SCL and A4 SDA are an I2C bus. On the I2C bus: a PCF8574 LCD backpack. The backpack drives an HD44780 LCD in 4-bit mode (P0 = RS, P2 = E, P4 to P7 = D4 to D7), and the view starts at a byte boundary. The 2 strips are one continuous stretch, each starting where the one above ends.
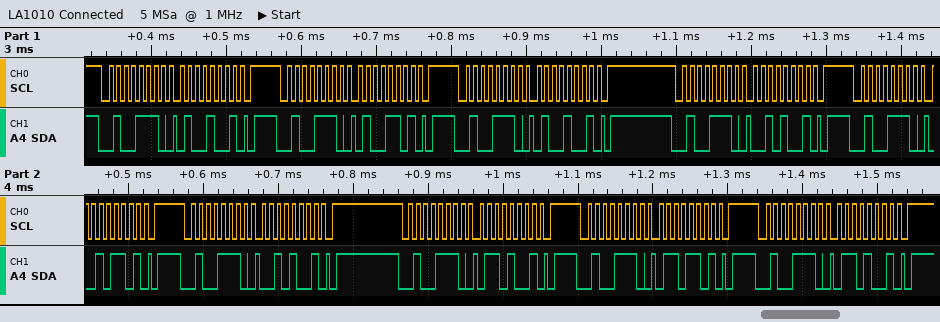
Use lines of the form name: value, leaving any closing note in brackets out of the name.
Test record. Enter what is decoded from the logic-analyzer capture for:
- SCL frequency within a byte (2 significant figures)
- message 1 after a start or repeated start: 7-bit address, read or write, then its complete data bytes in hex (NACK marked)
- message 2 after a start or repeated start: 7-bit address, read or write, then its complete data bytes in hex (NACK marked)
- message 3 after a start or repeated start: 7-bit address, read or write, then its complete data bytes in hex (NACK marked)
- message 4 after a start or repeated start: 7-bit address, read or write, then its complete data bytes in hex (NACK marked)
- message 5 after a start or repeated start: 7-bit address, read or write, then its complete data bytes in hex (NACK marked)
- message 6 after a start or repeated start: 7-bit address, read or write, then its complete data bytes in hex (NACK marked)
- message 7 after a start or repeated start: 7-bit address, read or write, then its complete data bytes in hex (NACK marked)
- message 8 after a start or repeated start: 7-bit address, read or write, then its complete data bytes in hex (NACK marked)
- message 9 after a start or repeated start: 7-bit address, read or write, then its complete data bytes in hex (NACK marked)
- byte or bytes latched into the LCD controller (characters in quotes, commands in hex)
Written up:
SCL frequency within a byte: 100 kHz
message 1 after a start or repeated start: 7-bit address, read or write, then its complete data bytes in hex: 0x27 write: 49
message 2 after a start or repeated start: 7-bit address, read or write, then its complete data bytes in hex: 0x27 write: 4D
message 3 after a start or repeated start: 7-bit address, read or write, then its complete data bytes in hex: 0x27 write: 49
message 4 after a start or repeated start: 7-bit address, read or write, then its complete data bytes in hex: 0x27 write: 29
message 5 after a start or repeated start: 7-bit address, read or write, then its complete data bytes in hex: 0x27 write: 2D
message 6 after a start or repeated start: 7-bit address, read or write, then its complete data bytes in hex: 0x27 write: 29
message 7 after a start or repeated start: 7-bit address, read or write, then its complete data bytes in hex: 0x27 write: 69
message 8 after a start or repeated start: 7-bit address, read or write, then its complete data bytes in hex: 0x27 write: 6D
message 9 after a start or repeated start: 7-bit address, read or write, then its complete data bytes in hex: 0x27 write: 69
byte or bytes latched into the LCD controller: 'B'
